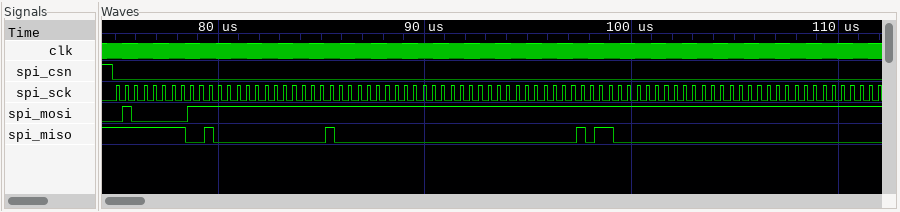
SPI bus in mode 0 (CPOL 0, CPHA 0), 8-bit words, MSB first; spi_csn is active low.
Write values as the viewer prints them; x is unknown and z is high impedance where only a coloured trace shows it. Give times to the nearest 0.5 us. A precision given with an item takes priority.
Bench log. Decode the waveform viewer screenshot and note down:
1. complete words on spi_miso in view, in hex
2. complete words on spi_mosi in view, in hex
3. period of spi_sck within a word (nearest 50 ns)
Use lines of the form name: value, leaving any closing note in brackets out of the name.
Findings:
complete words on spi_miso in view, in hex: FF, 20, 01, 00, 00, 00, 2C, 00, 00, 00
complete words on spi_mosi in view, in hex: 40, FF, FF, FF, FF, FF, FF, FF, FF, FF
period of spi_sck within a word: 450 ns
